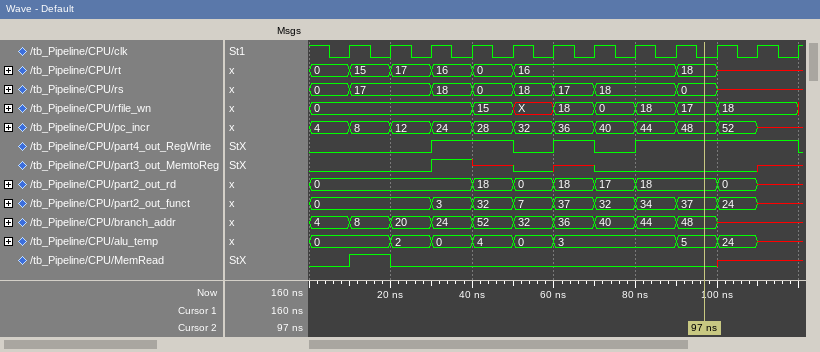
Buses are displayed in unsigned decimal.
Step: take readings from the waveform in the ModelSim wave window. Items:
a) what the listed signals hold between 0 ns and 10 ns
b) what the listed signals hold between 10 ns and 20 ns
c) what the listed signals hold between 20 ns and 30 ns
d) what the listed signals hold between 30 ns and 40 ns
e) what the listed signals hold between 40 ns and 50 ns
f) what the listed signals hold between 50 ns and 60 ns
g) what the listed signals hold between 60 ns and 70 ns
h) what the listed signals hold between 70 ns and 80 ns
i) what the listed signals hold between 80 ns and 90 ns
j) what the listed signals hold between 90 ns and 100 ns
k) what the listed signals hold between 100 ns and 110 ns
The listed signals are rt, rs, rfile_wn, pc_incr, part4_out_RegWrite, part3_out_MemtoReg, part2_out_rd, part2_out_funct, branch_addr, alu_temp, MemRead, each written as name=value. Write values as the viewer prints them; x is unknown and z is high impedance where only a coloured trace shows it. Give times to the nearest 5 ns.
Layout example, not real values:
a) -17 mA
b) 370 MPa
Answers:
a) rt=0, rs=0, rfile_wn=0, pc_incr=4, part4_out_RegWrite=0, part3_out_MemtoReg=0, part2_out_rd=0, part2_out_funct=0, branch_addr=4, alu_temp=0, MemRead=0
b) rt=15, rs=17, rfile_wn=0, pc_incr=8, part4_out_RegWrite=0, part3_out_MemtoReg=0, part2_out_rd=0, part2_out_funct=0, branch_addr=8, alu_temp=0, MemRead=1
c) rt=17, rs=17, rfile_wn=0, pc_incr=12, part4_out_RegWrite=0, part3_out_MemtoReg=0, part2_out_rd=0, part2_out_funct=0, branch_addr=20, alu_temp=2, MemRead=0
d) rt=16, rs=18, rfile_wn=0, pc_incr=24, part4_out_RegWrite=1, part3_out_MemtoReg=1, part2_out_rd=0, part2_out_funct=3, branch_addr=24, alu_temp=0, MemRead=0
e) rt=0, rs=0, rfile_wn=15, pc_incr=28, part4_out_RegWrite=1, part3_out_MemtoReg=x, part2_out_rd=18, part2_out_funct=32, branch_addr=52, alu_temp=4, MemRead=0
f) rt=16, rs=18, rfile_wn=X, pc_incr=32, part4_out_RegWrite=0, part3_out_MemtoReg=0, part2_out_rd=0, part2_out_funct=7, branch_addr=32, alu_temp=0, MemRead=0
g) rt=16, rs=17, rfile_wn=18, pc_incr=36, part4_out_RegWrite=1, part3_out_MemtoReg=x, part2_out_rd=18, part2_out_funct=37, branch_addr=36, alu_temp=3, MemRead=0
h) rt=16, rs=18, rfile_wn=0, pc_incr=40, part4_out_RegWrite=0, part3_out_MemtoReg=0, part2_out_rd=17, part2_out_funct=32, branch_addr=40, alu_temp=3, MemRead=0
i) rt=16, rs=18, rfile_wn=18, pc_incr=44, part4_out_RegWrite=1, part3_out_MemtoReg=0, part2_out_rd=18, part2_out_funct=34, branch_addr=44, alu_temp=3, MemRead=0
j) rt=18, rs=0, rfile_wn=17, pc_incr=48, part4_out_RegWrite=1, part3_out_MemtoReg=0, part2_out_rd=18, part2_out_funct=37, branch_addr=48, alu_temp=5, MemRead=0
k) rt=x, rs=x, rfile_wn=18, pc_incr=52, part4_out_RegWrite=1, part3_out_MemtoReg=0, part2_out_rd=0, part2_out_funct=24, branch_addr=x, alu_temp=24, MemRead=x
